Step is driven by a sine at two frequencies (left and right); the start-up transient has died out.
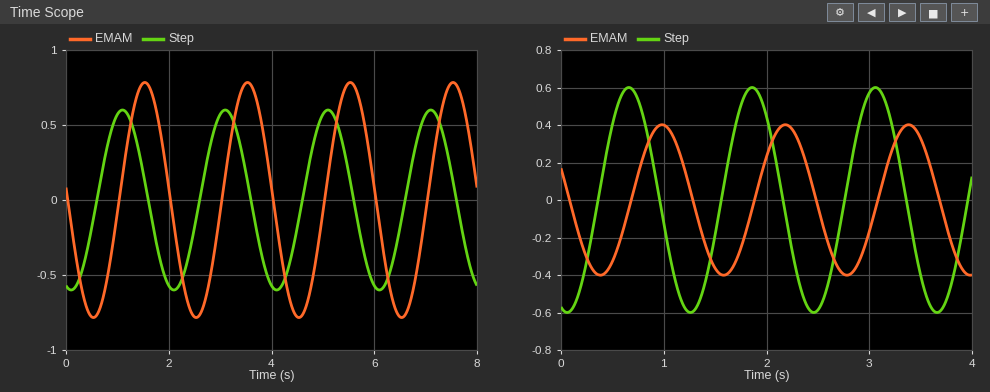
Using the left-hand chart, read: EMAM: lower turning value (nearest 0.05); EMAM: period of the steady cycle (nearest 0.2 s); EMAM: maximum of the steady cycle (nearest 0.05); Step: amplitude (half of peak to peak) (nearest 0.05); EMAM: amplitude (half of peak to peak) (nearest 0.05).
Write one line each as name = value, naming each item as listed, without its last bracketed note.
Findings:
EMAM: lower turning value = -0.80
EMAM: period of the steady cycle = 2.0 s
EMAM: maximum of the steady cycle = 0.80
Step: amplitude (half of peak to peak) = 0.60
EMAM: amplitude (half of peak to peak) = 0.80
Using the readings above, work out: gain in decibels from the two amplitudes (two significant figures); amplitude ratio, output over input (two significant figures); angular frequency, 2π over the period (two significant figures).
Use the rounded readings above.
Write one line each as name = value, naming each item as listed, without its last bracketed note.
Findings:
gain in decibels from the two amplitudes = 2.5 dB
amplitude ratio, output over input = 1.3
angular frequency, 2π over the period = 3.1 rad/s
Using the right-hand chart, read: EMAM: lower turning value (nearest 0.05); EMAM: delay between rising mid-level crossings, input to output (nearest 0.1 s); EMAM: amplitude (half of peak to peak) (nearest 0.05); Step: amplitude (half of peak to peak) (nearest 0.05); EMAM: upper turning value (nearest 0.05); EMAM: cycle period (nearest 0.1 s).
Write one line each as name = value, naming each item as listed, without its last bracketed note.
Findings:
EMAM: lower turning value = -0.40
EMAM: delay between rising mid-level crossings, input to output = 0.3 s
EMAM: amplitude (half of peak to peak) = 0.40
Step: amplitude (half of peak to peak) = 0.60
EMAM: upper turning value = 0.40
EMAM: cycle period = 1.2 s
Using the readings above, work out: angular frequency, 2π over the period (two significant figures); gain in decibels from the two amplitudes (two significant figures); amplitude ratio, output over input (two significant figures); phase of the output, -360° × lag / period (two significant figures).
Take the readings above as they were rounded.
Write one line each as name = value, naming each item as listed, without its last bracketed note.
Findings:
angular frequency, 2π over the period = 5.2 rad/s
gain in decibels from the two amplitudes = -3.5 dB
amplitude ratio, output over input = 0.67
phase of the output, -360° × lag / period = -90°
